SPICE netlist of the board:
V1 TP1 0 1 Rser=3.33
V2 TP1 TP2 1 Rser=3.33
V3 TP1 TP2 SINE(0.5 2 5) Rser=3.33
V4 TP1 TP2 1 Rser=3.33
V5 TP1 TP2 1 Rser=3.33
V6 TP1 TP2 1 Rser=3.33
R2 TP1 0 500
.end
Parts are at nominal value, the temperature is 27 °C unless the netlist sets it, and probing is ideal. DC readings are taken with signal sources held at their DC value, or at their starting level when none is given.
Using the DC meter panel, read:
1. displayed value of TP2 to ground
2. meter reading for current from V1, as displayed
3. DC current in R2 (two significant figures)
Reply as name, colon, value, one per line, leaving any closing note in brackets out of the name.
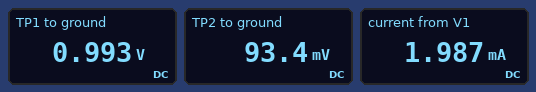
displayed value of TP2 to ground: 93.4 mV
meter reading for current from V1, as displayed: 1.987 mA
DC current in R2: 2.0 mA
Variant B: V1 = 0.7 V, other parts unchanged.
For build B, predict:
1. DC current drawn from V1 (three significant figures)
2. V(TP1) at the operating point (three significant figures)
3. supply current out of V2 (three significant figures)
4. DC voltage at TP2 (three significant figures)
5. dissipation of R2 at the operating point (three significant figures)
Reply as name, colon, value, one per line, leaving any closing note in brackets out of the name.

DC current drawn from V1: 1.39 mA
V(TP1) at the operating point: 695 mV
supply current out of V2: 30.0 mA
DC voltage at TP2: -205 mV
dissipation of R2 at the operating point: 967 µW
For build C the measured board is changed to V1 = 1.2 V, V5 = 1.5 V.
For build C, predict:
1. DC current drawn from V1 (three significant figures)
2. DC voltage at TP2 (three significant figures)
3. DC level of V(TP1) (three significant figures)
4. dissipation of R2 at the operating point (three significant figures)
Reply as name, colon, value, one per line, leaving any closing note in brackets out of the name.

DC current drawn from V1: 2.38 mA
DC voltage at TP2: 192 mV
DC level of V(TP1): 1.19 V
dissipation of R2 at the operating point: 2.84 mW
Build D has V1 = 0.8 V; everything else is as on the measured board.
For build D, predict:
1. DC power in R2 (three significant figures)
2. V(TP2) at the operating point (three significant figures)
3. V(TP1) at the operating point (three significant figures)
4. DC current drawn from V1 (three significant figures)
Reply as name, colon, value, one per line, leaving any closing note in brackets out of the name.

DC power in R2: 1.26 mW
V(TP2) at the operating point: -105 mV
V(TP1) at the operating point: 795 mV
DC current drawn from V1: 1.59 mA
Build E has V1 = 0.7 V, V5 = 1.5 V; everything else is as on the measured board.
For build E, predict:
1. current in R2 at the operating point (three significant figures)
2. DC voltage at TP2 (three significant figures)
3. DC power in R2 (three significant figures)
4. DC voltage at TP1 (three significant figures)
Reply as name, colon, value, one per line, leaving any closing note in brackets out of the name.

current in R2 at the operating point: 1.39 mA
DC voltage at TP2: -305 mV
DC power in R2: 967 µW
DC voltage at TP1: 695 mV
